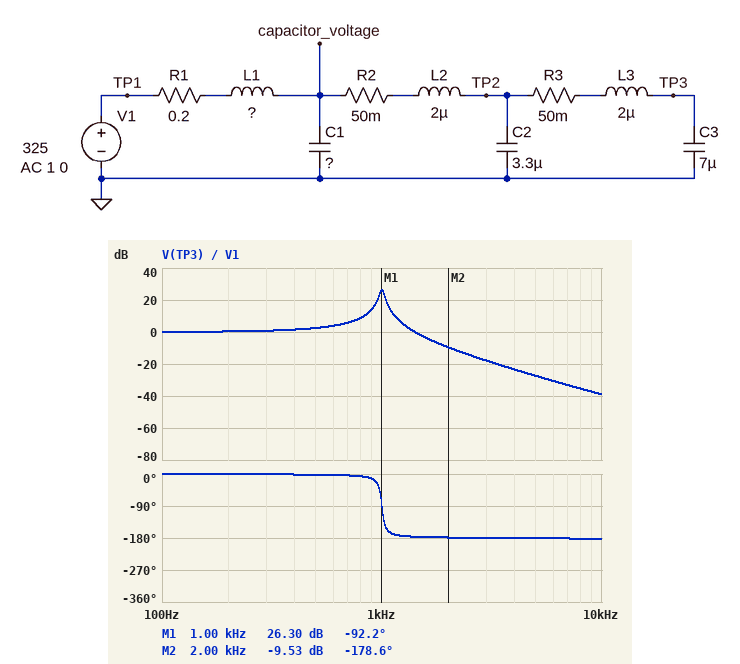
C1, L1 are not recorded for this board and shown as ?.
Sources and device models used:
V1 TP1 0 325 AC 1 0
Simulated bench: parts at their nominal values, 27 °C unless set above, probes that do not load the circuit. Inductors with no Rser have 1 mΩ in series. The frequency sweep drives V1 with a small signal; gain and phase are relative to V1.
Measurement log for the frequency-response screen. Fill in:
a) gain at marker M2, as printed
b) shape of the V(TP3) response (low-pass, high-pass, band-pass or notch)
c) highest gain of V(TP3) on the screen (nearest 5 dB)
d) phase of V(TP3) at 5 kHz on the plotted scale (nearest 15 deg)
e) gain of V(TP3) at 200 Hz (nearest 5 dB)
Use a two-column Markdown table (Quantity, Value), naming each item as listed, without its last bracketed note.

| Quantity | Value |
|---|---|
| gain at marker M2, as printed | -9.53 dB |
| shape of the V(TP3) response | low-pass |
| highest gain of V(TP3) on the screen | 25 dB |
| phase of V(TP3) at 5 kHz on the plotted scale | -180 deg |
| gain of V(TP3) at 200 Hz | 0 dB |
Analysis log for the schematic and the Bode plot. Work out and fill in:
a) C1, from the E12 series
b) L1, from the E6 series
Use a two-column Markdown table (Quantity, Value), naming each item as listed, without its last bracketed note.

| Quantity | Value |
|---|---|
| C1, from the E12 series | 27 µF |
| L1, from the E6 series | 680 µH |
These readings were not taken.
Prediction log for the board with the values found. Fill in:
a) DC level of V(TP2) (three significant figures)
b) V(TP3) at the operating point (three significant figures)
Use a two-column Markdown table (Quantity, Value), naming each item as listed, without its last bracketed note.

| Quantity | Value |
|---|---|
| DC level of V(TP2) | 325 V |
| V(TP3) at the operating point | 325 V |
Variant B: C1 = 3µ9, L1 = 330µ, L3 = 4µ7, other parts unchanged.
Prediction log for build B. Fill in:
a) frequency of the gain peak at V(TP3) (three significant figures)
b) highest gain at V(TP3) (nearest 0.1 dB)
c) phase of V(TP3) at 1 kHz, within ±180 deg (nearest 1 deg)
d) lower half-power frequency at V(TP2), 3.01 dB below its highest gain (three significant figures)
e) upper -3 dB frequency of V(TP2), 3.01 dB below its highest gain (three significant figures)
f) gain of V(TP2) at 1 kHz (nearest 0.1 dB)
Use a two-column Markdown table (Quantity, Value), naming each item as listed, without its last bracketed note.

| Quantity | Value |
|---|---|
| frequency of the gain peak at V(TP3) | 2.32 kHz |
| highest gain at V(TP3) | 26.1 dB |
| phase of V(TP3) at 1 kHz, within ±180 deg | -2 deg |
| lower half-power frequency at V(TP2), 3.01 dB below its highest gain | 2.26 kHz |
| upper -3 dB frequency of V(TP2), 3.01 dB below its highest gain | 2.37 kHz |
| gain of V(TP2) at 1 kHz | 1.8 dB |
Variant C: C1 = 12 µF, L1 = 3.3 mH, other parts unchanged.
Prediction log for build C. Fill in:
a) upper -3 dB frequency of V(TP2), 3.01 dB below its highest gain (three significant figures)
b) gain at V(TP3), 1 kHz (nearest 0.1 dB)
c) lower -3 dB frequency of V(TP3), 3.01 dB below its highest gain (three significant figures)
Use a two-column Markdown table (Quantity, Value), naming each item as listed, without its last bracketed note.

| Quantity | Value |
|---|---|
| upper -3 dB frequency of V(TP2), 3.01 dB below its highest gain | 592 Hz |
| gain at V(TP3), 1 kHz | -5.6 dB |
| lower -3 dB frequency of V(TP3), 3.01 dB below its highest gain | 581 Hz |
